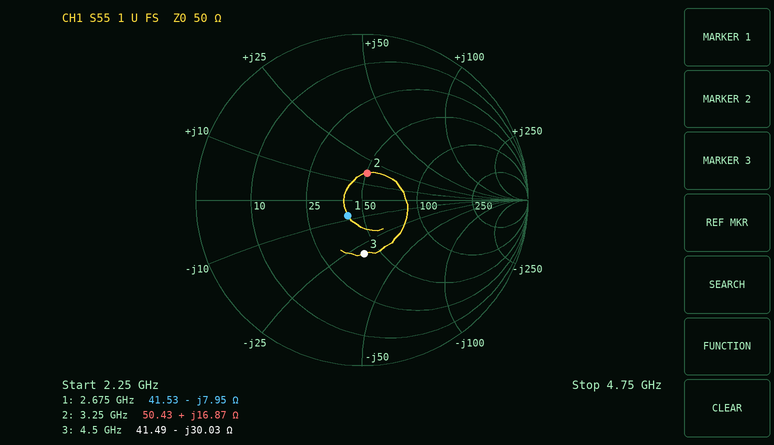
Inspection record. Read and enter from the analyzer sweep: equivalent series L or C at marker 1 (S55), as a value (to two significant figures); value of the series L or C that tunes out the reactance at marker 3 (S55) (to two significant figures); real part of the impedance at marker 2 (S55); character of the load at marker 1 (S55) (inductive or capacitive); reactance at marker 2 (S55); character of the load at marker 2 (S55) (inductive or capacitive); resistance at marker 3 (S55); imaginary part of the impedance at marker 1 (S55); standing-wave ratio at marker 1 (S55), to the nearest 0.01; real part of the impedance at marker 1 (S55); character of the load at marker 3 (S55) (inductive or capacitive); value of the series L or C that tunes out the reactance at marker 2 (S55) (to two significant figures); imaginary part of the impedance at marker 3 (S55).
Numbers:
7.5 pF
1.1 nH
50.43 Ω
capacitive
+16.87 Ω
inductive
41.49 Ω
-7.95 Ω
1.29
41.53 Ω
capacitive
2.9 pF
-30.03 Ω
